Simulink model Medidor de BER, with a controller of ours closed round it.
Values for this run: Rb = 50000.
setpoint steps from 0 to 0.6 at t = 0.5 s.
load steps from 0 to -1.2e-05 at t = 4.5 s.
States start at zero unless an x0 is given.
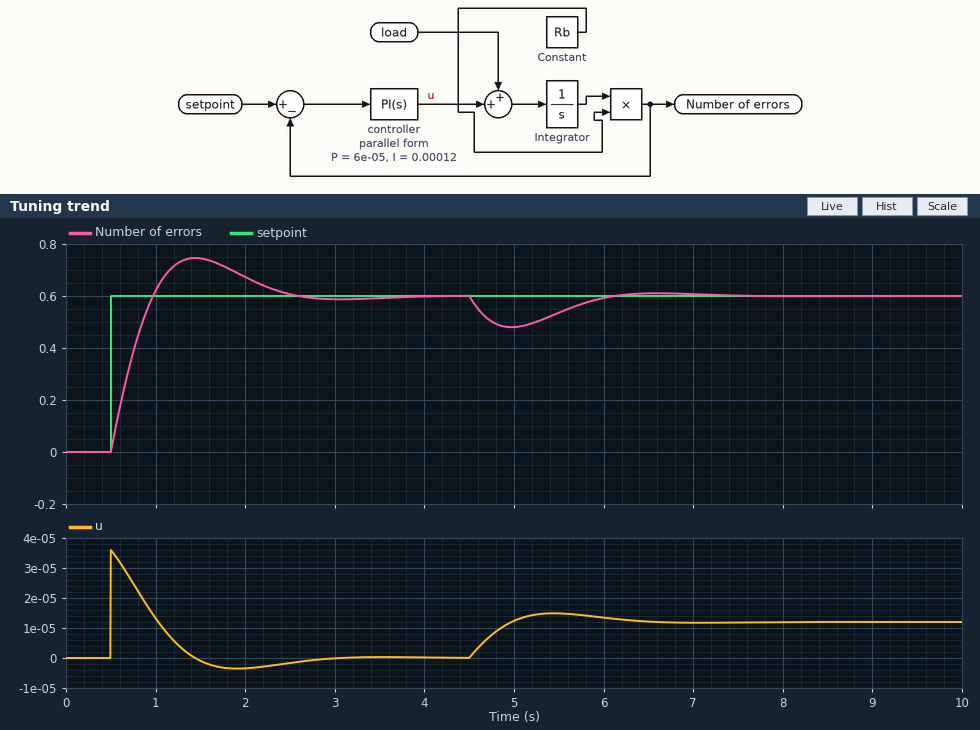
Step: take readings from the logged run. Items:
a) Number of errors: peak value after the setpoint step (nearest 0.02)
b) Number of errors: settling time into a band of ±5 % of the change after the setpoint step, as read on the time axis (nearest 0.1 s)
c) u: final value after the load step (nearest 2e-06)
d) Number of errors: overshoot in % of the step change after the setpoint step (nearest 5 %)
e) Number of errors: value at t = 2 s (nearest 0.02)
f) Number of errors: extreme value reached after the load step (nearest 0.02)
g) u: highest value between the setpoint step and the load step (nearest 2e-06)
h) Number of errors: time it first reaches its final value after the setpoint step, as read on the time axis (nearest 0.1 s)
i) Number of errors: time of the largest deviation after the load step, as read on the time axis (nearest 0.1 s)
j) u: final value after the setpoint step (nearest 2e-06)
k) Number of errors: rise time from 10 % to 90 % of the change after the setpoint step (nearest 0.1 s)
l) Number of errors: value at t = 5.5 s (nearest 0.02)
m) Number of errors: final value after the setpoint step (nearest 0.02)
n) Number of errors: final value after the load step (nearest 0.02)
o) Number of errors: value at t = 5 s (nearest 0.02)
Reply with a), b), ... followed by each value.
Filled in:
a) 0.74
b) 2.3 s
c) 0.000012
d) 25 %
e) 0.68
f) 0.48
g) 0.000036
h) 1.0 s
i) 5.0 s
j) 0.000000
k) 0.4 s
l) 0.54
m) 0.60
n) 0.60
o) 0.48
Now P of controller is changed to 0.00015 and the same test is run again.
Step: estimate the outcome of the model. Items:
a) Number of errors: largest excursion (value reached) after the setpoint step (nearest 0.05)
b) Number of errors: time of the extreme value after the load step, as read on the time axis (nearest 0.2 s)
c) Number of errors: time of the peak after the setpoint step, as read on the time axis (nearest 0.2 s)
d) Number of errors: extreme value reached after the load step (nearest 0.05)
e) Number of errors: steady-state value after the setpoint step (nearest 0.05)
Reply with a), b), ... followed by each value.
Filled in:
a) 0.65
b) 4.8 s
c) 1.2 s
d) 0.55
e) 0.60
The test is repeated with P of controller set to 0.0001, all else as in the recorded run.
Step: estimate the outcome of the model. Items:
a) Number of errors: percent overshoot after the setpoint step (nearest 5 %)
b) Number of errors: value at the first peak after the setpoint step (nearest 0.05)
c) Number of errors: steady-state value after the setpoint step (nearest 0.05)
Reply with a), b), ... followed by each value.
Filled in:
a) 15 %
b) 0.70
c) 0.60
